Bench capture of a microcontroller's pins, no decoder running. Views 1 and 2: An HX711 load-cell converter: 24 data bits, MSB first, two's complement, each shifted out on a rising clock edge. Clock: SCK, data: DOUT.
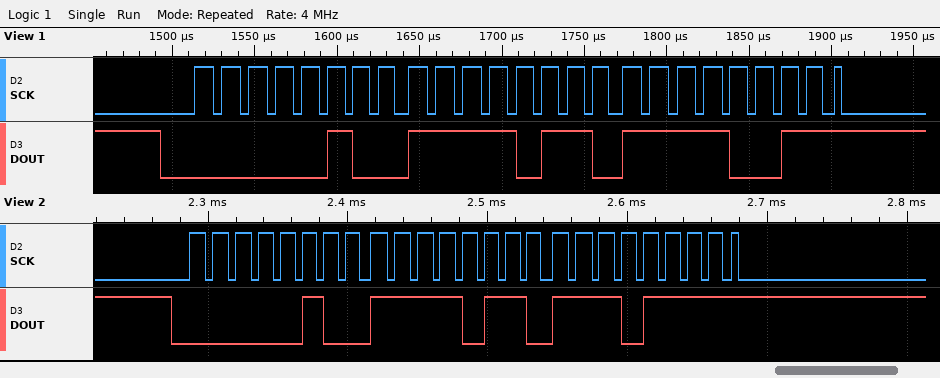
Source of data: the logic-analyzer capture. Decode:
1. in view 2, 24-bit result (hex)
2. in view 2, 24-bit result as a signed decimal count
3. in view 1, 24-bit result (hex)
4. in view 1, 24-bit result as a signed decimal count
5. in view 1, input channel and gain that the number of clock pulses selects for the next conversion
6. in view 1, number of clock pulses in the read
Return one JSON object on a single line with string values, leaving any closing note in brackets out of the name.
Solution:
{"in view 2, 24-bit result": "0x04F6EF", "in view 2, 24-bit result as a signed decimal count": "325359", "in view 1, 24-bit result": "0x04F6F3", "in view 1, 24-bit result as a signed decimal count": "325363", "in view 1, input channel and gain that the number of clock pulses selects for the next conversion": "channel A, gain 128", "in view 1, number of clock pulses in the read": "25"}
